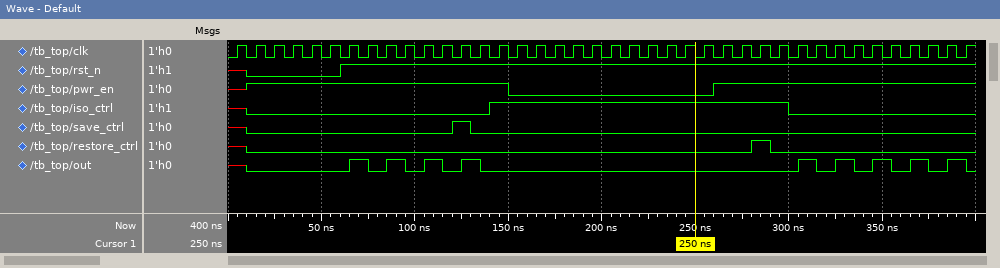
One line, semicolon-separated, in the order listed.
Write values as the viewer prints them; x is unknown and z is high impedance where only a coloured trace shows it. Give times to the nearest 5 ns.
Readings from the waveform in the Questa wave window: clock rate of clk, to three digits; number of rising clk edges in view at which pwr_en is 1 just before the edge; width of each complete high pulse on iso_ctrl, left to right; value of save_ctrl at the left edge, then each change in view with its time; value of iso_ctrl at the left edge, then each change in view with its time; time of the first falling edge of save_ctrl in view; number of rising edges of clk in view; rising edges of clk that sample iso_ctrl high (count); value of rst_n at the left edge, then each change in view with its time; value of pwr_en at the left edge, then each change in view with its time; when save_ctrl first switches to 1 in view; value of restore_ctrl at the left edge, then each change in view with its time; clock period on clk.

100 MHz; 28; 160 ns; x, 0 at 10 ns, 1 at 120 ns, 0 at 130 ns; x, 0 at 10 ns, 1 at 140 ns, 0 at 300 ns; 130 ns; 40; 16; x, 0 at 10 ns, 1 at 60 ns; x, 1 at 10 ns, 0 at 150 ns, 1 at 260 ns; 120 ns; x, 0 at 10 ns, 1 at 280 ns, 0 at 290 ns; 10 ns
